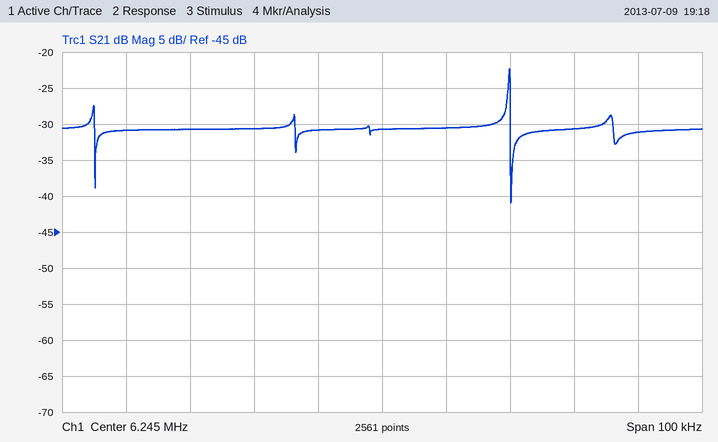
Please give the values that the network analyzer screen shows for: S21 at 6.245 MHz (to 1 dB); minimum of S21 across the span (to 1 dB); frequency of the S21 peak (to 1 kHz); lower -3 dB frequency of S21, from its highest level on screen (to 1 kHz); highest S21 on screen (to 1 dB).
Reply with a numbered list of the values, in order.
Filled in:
1. -31 dB
2. -41 dB
3. 6.265 MHz
4. 6.265 MHz
5. -22 dB
